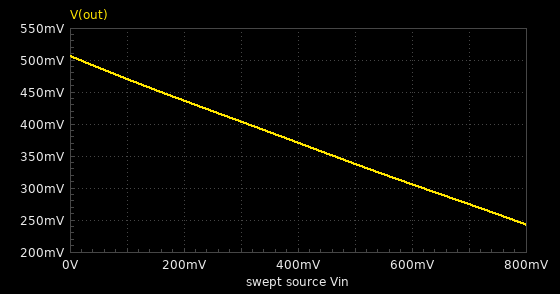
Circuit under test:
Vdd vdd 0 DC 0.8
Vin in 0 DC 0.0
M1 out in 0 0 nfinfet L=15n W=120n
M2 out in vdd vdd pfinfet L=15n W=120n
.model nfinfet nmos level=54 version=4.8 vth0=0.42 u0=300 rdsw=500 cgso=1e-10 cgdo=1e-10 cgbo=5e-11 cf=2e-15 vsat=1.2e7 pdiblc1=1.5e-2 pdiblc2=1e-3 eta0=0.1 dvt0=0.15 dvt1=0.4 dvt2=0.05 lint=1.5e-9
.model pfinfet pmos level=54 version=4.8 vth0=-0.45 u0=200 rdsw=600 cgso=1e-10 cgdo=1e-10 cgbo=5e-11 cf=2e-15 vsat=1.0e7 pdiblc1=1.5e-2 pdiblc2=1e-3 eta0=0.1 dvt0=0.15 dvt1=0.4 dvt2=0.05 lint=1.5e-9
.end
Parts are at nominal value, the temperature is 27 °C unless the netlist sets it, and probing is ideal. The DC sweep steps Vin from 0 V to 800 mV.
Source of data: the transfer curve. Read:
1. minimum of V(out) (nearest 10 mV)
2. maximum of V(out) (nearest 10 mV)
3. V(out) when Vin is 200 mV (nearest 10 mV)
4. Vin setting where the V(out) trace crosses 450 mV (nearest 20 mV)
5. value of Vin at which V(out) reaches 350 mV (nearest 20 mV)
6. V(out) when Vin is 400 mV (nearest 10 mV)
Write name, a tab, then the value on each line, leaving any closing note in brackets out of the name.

minimum of V(out)	240 mV
maximum of V(out)	510 mV
V(out) when Vin is 200 mV	440 mV
Vin setting where the V(out) trace crosses 450 mV	160 mV
value of Vin at which V(out) reaches 350 mV	460 mV
V(out) when Vin is 400 mV	370 mV
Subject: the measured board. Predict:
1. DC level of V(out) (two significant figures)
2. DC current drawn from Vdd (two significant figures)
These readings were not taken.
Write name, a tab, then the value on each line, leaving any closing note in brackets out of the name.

DC level of V(out)	510 mV
DC current drawn from Vdd	62 µA
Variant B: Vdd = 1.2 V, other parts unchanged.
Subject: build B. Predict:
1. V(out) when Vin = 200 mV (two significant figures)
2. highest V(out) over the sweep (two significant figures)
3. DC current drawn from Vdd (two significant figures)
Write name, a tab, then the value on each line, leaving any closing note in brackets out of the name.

V(out) when Vin = 200 mV	650 mV
highest V(out) over the sweep	690 mV
DC current drawn from Vdd	180 µA
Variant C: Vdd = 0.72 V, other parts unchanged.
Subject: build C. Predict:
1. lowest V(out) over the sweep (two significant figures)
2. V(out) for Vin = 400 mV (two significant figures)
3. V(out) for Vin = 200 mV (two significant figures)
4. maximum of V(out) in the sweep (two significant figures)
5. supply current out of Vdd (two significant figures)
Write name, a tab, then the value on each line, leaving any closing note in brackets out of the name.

lowest V(out) over the sweep	170 mV
V(out) for Vin = 400 mV	320 mV
V(out) for Vin = 200 mV	400 mV
maximum of V(out) in the sweep	480 mV
supply current out of Vdd	41 µA
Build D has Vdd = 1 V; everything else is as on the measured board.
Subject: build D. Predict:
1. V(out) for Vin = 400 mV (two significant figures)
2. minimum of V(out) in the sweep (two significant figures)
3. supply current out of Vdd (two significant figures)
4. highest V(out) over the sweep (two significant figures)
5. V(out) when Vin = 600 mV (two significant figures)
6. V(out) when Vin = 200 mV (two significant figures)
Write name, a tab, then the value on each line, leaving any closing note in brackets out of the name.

V(out) for Vin = 400 mV	490 mV
minimum of V(out) in the sweep	380 mV
supply current out of Vdd	120 µA
highest V(out) over the sweep	590 mV
V(out) when Vin = 600 mV	430 mV
V(out) when Vin = 200 mV	540 mV
